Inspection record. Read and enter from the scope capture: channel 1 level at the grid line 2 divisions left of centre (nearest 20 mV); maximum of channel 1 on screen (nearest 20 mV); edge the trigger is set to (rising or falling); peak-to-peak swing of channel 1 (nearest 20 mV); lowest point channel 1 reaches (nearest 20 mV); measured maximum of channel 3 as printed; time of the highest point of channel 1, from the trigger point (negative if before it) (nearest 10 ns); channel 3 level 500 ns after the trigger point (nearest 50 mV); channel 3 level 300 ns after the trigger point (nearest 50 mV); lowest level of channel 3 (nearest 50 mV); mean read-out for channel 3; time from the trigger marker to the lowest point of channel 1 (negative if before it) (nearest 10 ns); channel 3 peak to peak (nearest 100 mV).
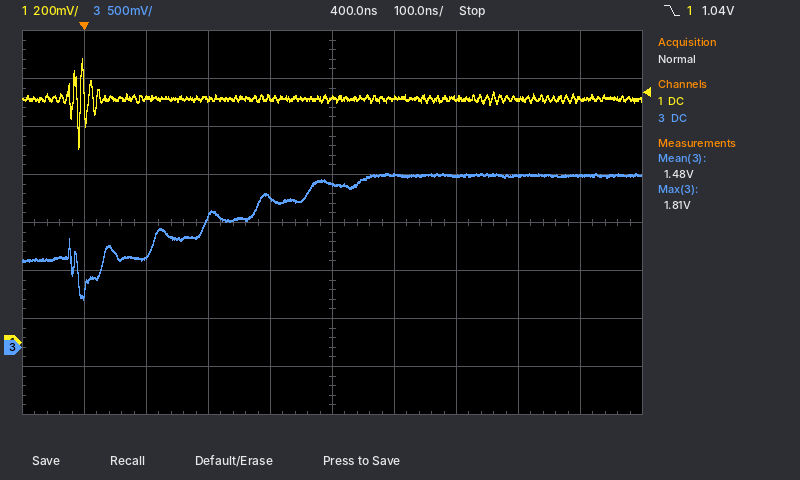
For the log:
1.02 V
1.18 V
falling
380 mV
800 mV
1.81 V
0 ns
1.80 V
1.55 V
500 mV
1.48 V
-10 ns
1.30 V
